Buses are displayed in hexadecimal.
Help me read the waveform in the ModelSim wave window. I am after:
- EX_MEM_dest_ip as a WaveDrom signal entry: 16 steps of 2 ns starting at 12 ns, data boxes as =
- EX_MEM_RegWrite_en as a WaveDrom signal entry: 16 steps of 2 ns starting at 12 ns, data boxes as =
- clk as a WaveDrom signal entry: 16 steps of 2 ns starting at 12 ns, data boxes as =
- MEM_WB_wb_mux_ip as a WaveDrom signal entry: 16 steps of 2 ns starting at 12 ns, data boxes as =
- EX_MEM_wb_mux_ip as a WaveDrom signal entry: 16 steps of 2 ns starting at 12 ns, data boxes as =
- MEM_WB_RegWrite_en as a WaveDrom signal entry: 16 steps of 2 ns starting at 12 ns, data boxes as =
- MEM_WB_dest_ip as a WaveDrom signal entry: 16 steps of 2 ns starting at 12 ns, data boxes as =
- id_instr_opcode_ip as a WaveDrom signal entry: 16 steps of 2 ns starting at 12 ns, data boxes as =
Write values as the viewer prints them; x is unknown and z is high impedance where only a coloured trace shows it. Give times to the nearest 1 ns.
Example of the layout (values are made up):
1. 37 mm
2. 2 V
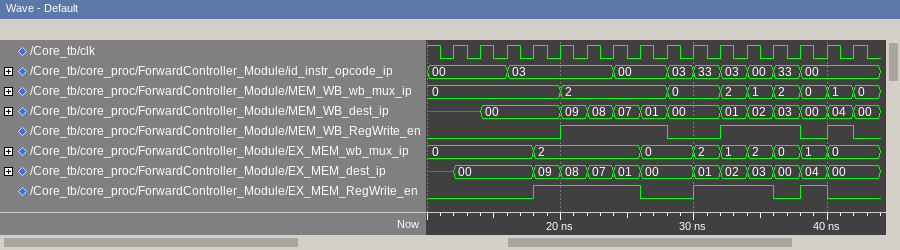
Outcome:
1. {name: 'EX_MEM_dest_ip', wave: '=..=====.======.', data: '00 09 08 07 01 00 01 02 03 00 04 00'}
2. {name: 'EX_MEM_RegWrite_en', wave: '0..1...0.1..010.'}
3. {name: 'clk', wave: 'p...............'}
4. {name: 'MEM_WB_wb_mux_ip', wave: '=...=...=.======', data: '0 2 0 2 1 2 0 1 0'}
5. {name: 'EX_MEM_wb_mux_ip', wave: '=..=...=.======.', data: '0 2 0 2 1 2 0 1 0'}
6. {name: 'MEM_WB_RegWrite_en', wave: '0...1...0.1..010'}
7. {name: 'MEM_WB_dest_ip', wave: 'z=..=====.======', data: '00 09 08 07 01 00 01 02 03 00 04 00'}
8. {name: 'id_instr_opcode_ip', wave: '=.=...=.======..', data: '00 03 00 03 33 03 00 33 00'}
